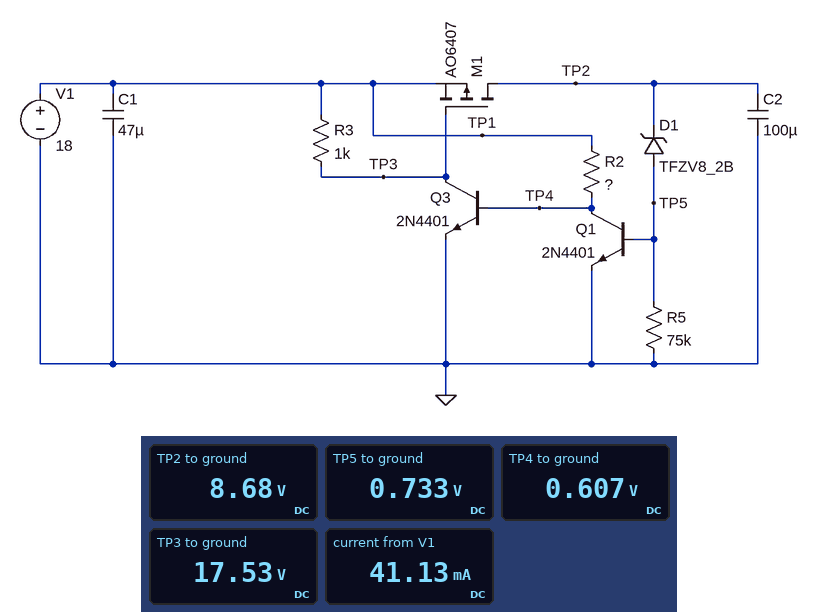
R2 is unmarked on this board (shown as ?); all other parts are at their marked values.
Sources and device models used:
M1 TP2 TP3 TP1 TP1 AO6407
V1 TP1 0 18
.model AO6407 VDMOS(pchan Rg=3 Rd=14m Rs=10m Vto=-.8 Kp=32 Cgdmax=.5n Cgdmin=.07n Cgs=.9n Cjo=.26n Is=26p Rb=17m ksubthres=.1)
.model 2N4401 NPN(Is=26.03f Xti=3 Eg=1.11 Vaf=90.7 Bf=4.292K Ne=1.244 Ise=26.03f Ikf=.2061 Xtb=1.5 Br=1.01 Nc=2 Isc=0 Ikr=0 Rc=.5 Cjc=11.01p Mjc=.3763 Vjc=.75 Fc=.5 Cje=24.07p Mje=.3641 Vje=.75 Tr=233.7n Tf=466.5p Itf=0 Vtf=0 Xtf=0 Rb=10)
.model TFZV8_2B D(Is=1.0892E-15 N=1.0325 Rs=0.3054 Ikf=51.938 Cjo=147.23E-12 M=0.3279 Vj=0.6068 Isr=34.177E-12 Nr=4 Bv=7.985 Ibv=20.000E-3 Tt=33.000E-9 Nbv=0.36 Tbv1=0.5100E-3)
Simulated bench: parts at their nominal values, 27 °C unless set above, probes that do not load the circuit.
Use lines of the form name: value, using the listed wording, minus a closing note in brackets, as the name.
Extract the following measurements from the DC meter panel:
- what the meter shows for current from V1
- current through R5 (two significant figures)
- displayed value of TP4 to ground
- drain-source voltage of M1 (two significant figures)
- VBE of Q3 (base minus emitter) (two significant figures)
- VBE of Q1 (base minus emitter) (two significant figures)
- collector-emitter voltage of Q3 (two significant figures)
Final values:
what the meter shows for current from V1: 41.13 mA
current through R5: 9.8 µA
displayed value of TP4 to ground: 0.607 V
drain-source voltage of M1: -9.3 V
VBE of Q3 (base minus emitter): 610 mV
VBE of Q1 (base minus emitter): 730 mV
collector-emitter voltage of Q3: 18 V
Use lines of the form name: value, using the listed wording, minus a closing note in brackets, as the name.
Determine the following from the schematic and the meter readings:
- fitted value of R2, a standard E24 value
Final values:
fitted value of R2, a standard E24 value: 430 Ω
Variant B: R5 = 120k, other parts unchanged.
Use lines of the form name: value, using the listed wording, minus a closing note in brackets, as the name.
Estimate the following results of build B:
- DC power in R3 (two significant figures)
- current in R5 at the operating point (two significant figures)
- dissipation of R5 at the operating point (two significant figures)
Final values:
DC power in R3: 220 µW
current in R5 at the operating point: 6.1 µA
dissipation of R5 at the operating point: 4.5 µW
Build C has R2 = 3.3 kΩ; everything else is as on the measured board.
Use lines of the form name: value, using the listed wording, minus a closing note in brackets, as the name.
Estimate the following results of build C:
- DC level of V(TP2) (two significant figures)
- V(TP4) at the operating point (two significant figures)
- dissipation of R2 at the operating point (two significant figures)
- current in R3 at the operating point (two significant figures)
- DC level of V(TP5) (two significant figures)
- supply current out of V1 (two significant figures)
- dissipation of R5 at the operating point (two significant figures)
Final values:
DC level of V(TP2): 8.6 V
V(TP4) at the operating point: 600 mV
dissipation of R2 at the operating point: 92 mW
current in R3 at the operating point: 390 µA
DC level of V(TP5): 670 mV
supply current out of V1: 5.7 mA
dissipation of R5 at the operating point: 6.1 µW
